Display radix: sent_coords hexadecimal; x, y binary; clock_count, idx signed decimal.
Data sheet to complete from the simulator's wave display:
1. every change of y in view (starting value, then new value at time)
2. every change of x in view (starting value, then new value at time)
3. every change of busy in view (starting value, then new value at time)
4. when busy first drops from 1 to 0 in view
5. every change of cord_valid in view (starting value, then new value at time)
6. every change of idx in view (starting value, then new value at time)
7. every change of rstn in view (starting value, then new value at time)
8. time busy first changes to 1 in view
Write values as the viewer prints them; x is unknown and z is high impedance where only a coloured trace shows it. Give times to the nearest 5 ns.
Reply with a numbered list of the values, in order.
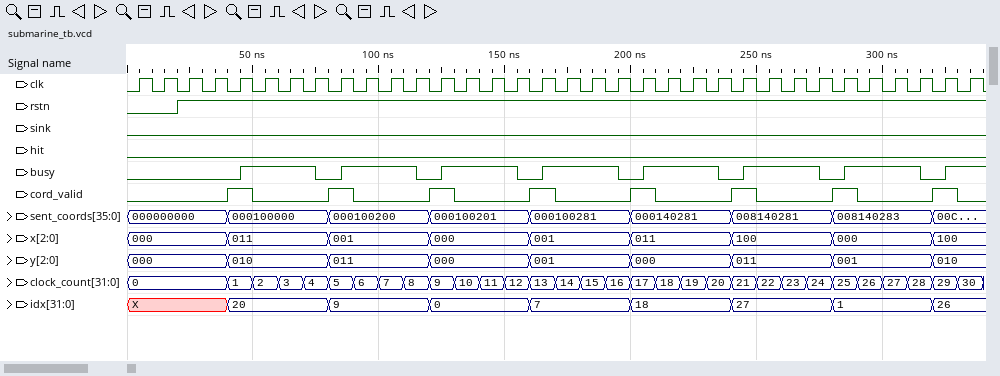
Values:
1. 000, 010 at 40 ns, 011 at 80 ns, 000 at 120 ns, 001 at 160 ns, 000 at 200 ns, 011 at 240 ns, 001 at 280 ns, 010 at 320 ns
2. 000, 011 at 40 ns, 001 at 80 ns, 000 at 120 ns, 001 at 160 ns, 011 at 200 ns, 100 at 240 ns, 000 at 280 ns, 100 at 320 ns
3. 0, 1 at 45 ns, 0 at 75 ns, 1 at 85 ns, 0 at 115 ns, 1 at 125 ns, 0 at 155 ns, 1 at 165 ns, 0 at 195 ns, 1 at 205 ns, 0 at 235 ns, 1 at 245 ns, 0 at 275 ns, 1 at 285 ns, 0 at 315 ns, 1 at 325 ns
4. 75 ns
5. 0, 1 at 40 ns, 0 at 50 ns, 1 at 80 ns, 0 at 90 ns, 1 at 120 ns, 0 at 130 ns, 1 at 160 ns, 0 at 170 ns, 1 at 200 ns, 0 at 210 ns, 1 at 240 ns, 0 at 250 ns, 1 at 280 ns, 0 at 290 ns, 1 at 320 ns, 0 at 330 ns
6. X, 20 at 40 ns, 9 at 80 ns, 0 at 120 ns, 7 at 160 ns, 18 at 200 ns, 27 at 240 ns, 1 at 280 ns, 26 at 320 ns
7. 0, 1 at 20 ns
8. 45 ns
